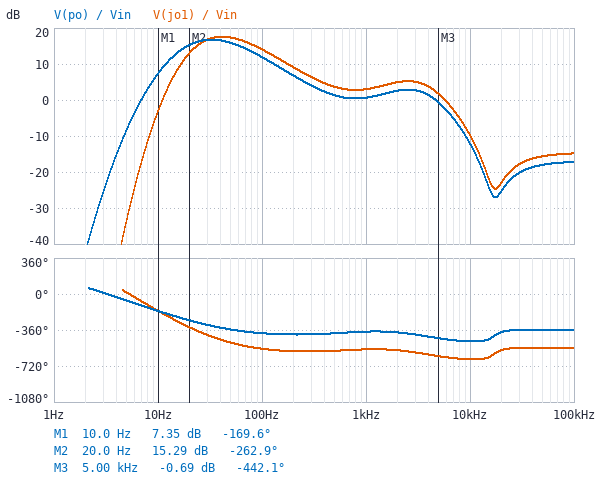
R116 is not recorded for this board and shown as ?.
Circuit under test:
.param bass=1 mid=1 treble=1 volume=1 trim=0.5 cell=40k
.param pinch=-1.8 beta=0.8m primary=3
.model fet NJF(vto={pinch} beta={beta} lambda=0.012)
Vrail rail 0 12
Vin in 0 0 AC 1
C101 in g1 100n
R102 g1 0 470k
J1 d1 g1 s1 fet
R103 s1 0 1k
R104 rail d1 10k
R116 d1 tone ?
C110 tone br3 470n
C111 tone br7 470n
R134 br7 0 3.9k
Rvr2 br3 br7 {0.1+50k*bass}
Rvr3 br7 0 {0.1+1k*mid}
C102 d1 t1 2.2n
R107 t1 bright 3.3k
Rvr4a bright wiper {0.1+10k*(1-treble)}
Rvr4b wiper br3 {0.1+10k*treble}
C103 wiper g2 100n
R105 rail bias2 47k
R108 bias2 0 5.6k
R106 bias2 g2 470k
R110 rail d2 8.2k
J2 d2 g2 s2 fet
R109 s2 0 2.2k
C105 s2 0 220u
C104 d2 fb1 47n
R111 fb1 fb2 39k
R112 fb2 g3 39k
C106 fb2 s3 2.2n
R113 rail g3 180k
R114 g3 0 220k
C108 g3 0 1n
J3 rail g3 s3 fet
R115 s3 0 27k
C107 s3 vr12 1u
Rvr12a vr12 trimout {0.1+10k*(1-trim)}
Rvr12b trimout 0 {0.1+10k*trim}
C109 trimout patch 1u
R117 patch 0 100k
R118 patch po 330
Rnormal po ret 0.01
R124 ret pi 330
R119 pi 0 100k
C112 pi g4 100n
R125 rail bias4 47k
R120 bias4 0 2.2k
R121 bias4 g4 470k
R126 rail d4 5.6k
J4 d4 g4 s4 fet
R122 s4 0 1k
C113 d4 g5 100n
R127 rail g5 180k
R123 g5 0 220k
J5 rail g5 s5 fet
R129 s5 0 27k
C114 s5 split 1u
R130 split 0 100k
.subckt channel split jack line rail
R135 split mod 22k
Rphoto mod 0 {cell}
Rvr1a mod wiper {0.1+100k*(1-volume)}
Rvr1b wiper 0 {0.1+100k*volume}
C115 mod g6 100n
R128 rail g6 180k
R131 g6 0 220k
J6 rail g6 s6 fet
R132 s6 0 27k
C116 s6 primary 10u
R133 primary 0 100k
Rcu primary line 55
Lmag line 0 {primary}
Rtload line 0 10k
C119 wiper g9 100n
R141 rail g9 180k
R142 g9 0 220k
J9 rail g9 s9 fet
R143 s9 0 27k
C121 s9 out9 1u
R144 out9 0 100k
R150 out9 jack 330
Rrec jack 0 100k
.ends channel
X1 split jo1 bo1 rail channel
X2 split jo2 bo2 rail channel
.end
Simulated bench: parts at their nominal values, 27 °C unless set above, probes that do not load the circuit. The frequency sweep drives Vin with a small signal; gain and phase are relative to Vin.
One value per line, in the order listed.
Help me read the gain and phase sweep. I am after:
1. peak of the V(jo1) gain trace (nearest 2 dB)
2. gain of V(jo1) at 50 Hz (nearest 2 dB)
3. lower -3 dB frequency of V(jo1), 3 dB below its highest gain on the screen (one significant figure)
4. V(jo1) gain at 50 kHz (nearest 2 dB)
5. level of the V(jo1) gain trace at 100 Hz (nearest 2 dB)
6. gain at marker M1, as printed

18 dB
18 dB
20 Hz
-16 dB
14 dB
7.35 dB
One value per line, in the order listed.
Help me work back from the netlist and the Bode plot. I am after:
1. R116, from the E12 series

3.3 kΩ
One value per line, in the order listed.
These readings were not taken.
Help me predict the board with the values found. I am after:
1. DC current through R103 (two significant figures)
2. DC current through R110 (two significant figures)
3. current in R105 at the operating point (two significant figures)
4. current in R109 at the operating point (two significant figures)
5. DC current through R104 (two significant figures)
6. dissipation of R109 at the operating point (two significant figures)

810 µA
920 µA
230 µA
920 µA
810 µA
1.9 mW
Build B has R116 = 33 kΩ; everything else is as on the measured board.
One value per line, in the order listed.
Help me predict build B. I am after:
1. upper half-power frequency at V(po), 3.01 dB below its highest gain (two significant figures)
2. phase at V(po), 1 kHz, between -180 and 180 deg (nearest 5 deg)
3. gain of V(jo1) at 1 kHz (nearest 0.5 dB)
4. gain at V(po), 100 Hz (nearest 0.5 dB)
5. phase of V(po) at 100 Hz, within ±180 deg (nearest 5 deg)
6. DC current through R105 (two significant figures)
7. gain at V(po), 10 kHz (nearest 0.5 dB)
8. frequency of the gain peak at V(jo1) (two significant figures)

4.6 kHz
35 deg
7.0 dB
1.5 dB
-35 deg
230 µA
-6.5 dB
2.6 kHz
